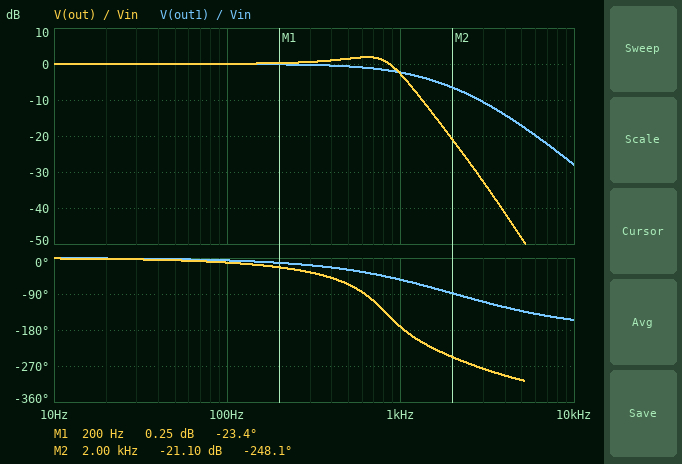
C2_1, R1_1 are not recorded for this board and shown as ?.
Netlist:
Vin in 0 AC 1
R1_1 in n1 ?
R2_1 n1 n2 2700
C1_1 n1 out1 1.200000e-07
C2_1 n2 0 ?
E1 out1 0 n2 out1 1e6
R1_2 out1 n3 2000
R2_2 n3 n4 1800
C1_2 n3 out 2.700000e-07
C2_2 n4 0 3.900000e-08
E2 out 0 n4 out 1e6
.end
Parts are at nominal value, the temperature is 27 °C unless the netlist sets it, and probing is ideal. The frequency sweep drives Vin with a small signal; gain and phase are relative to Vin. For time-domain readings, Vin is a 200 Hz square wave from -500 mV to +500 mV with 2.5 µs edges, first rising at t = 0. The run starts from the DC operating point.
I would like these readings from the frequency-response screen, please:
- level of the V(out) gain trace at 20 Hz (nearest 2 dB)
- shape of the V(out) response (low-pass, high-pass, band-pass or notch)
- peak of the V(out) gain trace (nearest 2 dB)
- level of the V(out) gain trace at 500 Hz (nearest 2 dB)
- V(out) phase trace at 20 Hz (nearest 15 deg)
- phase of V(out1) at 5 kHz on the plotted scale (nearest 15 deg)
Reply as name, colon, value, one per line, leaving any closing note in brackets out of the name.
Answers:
level of the V(out) gain trace at 20 Hz: 0 dB
shape of the V(out) response: low-pass
peak of the V(out) gain trace: 2 dB
level of the V(out) gain trace at 500 Hz: 2 dB
V(out) phase trace at 20 Hz: 0 deg
phase of V(out1) at 5 kHz on the plotted scale: -135 deg
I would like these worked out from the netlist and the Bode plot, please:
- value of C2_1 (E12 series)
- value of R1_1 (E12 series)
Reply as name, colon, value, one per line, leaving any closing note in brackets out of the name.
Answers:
value of C2_1: 56 nF
value of R1_1: 330 Ω
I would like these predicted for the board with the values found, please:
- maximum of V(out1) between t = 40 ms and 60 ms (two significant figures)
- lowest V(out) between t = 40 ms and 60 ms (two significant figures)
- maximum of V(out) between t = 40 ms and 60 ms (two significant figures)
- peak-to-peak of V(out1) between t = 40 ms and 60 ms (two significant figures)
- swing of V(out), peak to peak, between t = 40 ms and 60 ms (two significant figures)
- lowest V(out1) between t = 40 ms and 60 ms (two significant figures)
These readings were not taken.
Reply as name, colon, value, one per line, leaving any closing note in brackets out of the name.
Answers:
maximum of V(out1) between t = 40 ms and 60 ms: 500 mV
lowest V(out) between t = 40 ms and 60 ms: -710 mV
maximum of V(out) between t = 40 ms and 60 ms: 710 mV
peak-to-peak of V(out1) between t = 40 ms and 60 ms: 1.0 V
swing of V(out), peak to peak, between t = 40 ms and 60 ms: 1.4 V
lowest V(out1) between t = 40 ms and 60 ms: -500 mV
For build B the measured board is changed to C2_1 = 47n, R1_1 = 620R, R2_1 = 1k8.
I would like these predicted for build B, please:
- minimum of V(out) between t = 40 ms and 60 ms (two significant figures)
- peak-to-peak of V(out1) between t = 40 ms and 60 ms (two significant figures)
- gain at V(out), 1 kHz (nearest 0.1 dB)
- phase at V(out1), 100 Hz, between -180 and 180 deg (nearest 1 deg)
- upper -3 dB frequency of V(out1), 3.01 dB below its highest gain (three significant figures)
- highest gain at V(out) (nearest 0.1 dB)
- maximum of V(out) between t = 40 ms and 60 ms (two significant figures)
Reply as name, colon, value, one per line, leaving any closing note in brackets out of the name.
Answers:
minimum of V(out) between t = 40 ms and 60 ms: -780 mV
peak-to-peak of V(out1) between t = 40 ms and 60 ms: 1.1 V
gain at V(out), 1 kHz: -0.8 dB
phase at V(out1), 100 Hz, between -180 and 180 deg: -4 deg
upper -3 dB frequency of V(out1), 3.01 dB below its highest gain: 1.98 kHz
highest gain at V(out): 3.0 dB
maximum of V(out) between t = 40 ms and 60 ms: 780 mV
